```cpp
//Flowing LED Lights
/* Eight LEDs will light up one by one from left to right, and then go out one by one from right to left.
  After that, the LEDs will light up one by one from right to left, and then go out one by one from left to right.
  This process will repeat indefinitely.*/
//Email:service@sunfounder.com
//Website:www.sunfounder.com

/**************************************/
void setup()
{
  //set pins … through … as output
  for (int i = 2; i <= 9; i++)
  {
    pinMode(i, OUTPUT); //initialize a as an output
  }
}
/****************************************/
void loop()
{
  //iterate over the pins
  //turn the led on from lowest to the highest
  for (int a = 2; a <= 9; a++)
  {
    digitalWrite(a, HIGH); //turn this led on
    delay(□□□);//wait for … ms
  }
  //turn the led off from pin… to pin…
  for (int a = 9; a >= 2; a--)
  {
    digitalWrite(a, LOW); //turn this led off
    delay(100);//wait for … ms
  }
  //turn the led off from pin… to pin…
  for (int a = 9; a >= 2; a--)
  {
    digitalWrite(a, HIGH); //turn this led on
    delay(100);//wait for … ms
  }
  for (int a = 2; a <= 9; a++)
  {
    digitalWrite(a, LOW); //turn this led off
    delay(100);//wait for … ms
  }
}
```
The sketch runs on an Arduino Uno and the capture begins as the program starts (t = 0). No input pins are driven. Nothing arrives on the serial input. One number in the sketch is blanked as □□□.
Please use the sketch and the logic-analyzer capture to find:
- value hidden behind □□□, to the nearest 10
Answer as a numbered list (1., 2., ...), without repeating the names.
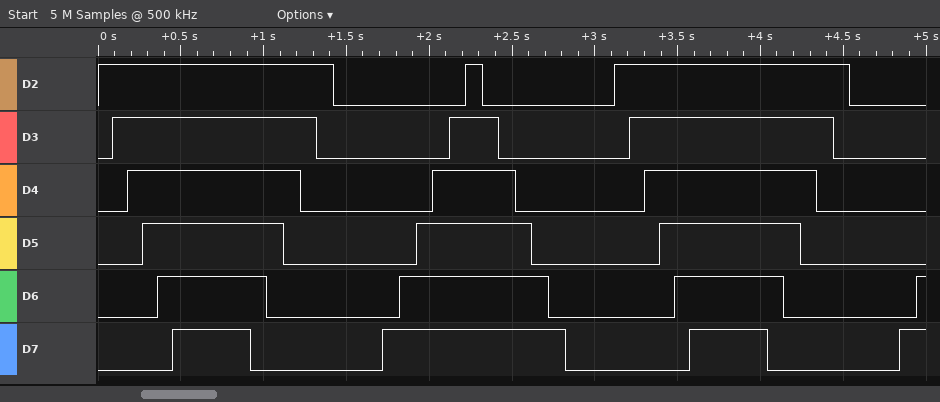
1. 90
